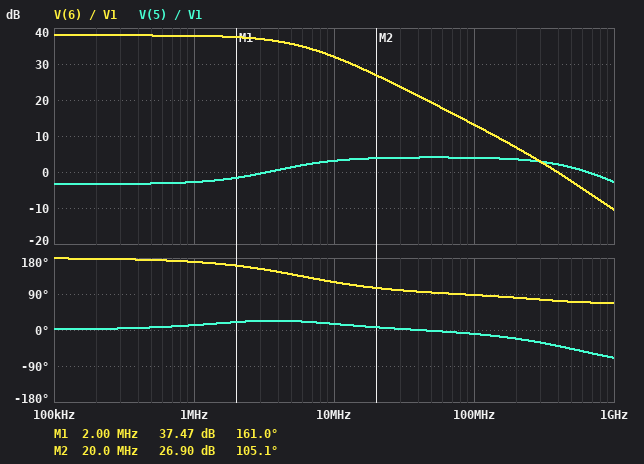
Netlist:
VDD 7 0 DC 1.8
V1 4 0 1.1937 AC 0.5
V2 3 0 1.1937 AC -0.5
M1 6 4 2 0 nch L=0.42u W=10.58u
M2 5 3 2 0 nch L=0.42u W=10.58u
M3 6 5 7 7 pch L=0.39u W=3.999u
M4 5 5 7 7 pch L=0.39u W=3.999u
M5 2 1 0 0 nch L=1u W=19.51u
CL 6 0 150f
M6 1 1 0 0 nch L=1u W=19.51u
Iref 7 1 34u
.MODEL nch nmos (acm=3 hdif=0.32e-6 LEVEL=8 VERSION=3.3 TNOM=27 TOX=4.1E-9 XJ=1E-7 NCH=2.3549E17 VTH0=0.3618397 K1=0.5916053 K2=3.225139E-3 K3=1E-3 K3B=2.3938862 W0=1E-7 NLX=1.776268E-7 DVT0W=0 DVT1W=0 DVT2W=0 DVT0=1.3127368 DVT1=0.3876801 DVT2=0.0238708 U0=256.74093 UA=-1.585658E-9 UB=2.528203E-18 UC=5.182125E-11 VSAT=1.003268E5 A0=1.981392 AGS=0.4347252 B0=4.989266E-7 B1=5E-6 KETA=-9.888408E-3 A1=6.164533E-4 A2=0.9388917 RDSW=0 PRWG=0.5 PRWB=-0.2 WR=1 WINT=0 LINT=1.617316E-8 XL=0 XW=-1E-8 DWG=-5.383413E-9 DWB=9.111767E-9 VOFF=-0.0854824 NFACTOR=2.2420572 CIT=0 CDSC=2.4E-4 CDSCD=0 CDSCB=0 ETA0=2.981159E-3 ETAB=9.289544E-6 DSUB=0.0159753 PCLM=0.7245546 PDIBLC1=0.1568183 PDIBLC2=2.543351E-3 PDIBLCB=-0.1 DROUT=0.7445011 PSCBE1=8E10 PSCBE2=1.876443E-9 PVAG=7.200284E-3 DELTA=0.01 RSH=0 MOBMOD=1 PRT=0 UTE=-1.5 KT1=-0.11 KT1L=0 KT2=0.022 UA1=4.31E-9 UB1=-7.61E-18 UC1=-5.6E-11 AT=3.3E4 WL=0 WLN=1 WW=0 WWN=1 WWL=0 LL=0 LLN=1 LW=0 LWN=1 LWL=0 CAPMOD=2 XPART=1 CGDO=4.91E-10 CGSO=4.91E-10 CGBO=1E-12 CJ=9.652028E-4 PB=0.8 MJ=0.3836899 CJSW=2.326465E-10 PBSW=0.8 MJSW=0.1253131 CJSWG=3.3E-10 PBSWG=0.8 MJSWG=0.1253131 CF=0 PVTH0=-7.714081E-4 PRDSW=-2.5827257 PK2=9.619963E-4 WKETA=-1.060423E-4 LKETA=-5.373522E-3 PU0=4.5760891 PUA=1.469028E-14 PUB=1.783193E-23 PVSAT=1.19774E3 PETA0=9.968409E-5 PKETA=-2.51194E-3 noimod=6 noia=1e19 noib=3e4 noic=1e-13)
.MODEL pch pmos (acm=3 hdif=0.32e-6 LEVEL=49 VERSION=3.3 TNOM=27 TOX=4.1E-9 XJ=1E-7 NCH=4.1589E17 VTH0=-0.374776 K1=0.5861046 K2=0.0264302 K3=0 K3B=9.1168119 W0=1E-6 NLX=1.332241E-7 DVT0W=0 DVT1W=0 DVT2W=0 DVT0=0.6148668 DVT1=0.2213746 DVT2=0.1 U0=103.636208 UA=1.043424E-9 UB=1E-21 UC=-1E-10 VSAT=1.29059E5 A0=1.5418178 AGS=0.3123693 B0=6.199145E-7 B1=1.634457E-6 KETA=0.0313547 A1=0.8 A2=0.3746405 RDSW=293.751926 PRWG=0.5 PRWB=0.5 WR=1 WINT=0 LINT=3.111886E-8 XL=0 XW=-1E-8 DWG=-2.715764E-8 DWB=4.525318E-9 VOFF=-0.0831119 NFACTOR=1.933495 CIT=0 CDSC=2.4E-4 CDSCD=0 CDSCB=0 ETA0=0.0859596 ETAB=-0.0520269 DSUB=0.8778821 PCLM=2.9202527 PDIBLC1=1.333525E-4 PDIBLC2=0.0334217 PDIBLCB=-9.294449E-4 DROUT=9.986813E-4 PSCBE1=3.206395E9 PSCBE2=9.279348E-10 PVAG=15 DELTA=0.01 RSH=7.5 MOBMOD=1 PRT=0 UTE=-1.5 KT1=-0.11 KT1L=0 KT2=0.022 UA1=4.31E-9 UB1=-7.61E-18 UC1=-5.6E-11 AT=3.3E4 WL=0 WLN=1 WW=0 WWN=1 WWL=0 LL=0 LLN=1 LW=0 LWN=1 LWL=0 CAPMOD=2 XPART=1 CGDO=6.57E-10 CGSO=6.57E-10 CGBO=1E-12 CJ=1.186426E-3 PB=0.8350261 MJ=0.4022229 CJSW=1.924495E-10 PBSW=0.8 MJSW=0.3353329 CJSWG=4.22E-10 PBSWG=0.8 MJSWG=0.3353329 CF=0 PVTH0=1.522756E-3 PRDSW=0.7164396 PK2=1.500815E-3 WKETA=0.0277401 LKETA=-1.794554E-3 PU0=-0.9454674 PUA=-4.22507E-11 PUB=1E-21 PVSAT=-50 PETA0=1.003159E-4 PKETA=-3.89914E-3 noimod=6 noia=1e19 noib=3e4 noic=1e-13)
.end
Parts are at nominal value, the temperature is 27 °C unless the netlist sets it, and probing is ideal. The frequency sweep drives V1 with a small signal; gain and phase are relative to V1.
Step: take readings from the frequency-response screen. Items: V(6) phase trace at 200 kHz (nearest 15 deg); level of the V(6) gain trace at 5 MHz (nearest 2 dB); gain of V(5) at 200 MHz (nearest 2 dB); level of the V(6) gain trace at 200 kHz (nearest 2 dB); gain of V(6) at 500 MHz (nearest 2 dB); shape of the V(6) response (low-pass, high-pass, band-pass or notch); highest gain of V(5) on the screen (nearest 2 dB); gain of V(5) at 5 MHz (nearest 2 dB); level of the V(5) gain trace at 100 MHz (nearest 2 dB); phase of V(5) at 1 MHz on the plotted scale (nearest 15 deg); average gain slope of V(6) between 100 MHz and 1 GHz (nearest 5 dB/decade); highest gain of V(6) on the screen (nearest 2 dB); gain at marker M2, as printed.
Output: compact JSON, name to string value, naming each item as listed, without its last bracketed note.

{"V(6) phase trace at 200 kHz": "180 deg", "level of the V(6) gain trace at 5 MHz": "36 dB", "gain of V(5) at 200 MHz": "4 dB", "level of the V(6) gain trace at 200 kHz": "38 dB", "gain of V(6) at 500 MHz": "-2 dB", "shape of the V(6) response": "low-pass", "highest gain of V(5) on the screen": "4 dB", "gain of V(5) at 5 MHz": "2 dB", "level of the V(5) gain trace at 100 MHz": "4 dB", "phase of V(5) at 1 MHz on the plotted scale": "15 deg", "average gain slope of V(6) between 100 MHz and 1 GHz": "-25 dB/decade", "highest gain of V(6) on the screen": "38 dB", "gain at marker M2, as printed": "26.90 dB"}
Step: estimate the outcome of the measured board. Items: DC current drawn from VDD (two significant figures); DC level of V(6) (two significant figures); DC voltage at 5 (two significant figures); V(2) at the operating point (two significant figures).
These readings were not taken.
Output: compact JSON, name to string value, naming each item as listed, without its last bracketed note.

{"DC current drawn from VDD": "68 µA", "DC level of V(6)": "1.1 V", "DC voltage at 5": "1.1 V", "V(2) at the operating point": "540 mV"}
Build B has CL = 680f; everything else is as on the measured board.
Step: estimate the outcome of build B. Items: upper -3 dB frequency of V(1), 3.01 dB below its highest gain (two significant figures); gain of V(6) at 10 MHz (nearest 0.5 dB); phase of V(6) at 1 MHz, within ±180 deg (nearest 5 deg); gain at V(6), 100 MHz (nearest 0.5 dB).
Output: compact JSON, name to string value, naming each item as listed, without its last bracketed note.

{"upper -3 dB frequency of V(1), 3.01 dB below its highest gain": "3.9 GHz", "gain of V(6) at 10 MHz": "21.0 dB", "phase of V(6) at 1 MHz, within ±180 deg": "145 deg", "gain at V(6), 100 MHz": "1.0 dB"}
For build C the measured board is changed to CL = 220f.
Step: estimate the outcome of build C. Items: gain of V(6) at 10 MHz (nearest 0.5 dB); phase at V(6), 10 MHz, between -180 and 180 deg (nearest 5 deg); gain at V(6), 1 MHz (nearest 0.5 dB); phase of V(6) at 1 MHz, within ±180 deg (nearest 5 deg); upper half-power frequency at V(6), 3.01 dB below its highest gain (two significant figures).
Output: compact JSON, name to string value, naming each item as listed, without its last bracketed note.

{"gain of V(6) at 10 MHz": "29.5 dB", "phase at V(6), 10 MHz, between -180 and 180 deg": "110 deg", "gain at V(6), 1 MHz": "37.5 dB", "phase of V(6) at 1 MHz, within ±180 deg": "165 deg", "upper half-power frequency at V(6), 3.01 dB below its highest gain": "4.2 MHz"}
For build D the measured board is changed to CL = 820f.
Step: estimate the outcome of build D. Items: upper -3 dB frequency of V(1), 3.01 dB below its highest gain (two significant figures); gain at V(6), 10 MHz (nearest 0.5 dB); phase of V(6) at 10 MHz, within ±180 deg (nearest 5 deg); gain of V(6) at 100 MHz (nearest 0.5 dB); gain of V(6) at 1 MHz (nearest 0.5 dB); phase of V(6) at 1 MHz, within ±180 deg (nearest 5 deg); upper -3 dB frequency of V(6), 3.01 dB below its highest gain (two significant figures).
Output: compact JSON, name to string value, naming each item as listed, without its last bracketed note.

{"upper -3 dB frequency of V(1), 3.01 dB below its highest gain": "3.9 GHz", "gain at V(6), 10 MHz": "19.5 dB", "phase of V(6) at 10 MHz, within ±180 deg": "95 deg", "gain of V(6) at 100 MHz": "-0.5 dB", "gain of V(6) at 1 MHz": "35.5 dB", "phase of V(6) at 1 MHz, within ±180 deg": "140 deg", "upper -3 dB frequency of V(6), 3.01 dB below its highest gain": "1.2 MHz"}
